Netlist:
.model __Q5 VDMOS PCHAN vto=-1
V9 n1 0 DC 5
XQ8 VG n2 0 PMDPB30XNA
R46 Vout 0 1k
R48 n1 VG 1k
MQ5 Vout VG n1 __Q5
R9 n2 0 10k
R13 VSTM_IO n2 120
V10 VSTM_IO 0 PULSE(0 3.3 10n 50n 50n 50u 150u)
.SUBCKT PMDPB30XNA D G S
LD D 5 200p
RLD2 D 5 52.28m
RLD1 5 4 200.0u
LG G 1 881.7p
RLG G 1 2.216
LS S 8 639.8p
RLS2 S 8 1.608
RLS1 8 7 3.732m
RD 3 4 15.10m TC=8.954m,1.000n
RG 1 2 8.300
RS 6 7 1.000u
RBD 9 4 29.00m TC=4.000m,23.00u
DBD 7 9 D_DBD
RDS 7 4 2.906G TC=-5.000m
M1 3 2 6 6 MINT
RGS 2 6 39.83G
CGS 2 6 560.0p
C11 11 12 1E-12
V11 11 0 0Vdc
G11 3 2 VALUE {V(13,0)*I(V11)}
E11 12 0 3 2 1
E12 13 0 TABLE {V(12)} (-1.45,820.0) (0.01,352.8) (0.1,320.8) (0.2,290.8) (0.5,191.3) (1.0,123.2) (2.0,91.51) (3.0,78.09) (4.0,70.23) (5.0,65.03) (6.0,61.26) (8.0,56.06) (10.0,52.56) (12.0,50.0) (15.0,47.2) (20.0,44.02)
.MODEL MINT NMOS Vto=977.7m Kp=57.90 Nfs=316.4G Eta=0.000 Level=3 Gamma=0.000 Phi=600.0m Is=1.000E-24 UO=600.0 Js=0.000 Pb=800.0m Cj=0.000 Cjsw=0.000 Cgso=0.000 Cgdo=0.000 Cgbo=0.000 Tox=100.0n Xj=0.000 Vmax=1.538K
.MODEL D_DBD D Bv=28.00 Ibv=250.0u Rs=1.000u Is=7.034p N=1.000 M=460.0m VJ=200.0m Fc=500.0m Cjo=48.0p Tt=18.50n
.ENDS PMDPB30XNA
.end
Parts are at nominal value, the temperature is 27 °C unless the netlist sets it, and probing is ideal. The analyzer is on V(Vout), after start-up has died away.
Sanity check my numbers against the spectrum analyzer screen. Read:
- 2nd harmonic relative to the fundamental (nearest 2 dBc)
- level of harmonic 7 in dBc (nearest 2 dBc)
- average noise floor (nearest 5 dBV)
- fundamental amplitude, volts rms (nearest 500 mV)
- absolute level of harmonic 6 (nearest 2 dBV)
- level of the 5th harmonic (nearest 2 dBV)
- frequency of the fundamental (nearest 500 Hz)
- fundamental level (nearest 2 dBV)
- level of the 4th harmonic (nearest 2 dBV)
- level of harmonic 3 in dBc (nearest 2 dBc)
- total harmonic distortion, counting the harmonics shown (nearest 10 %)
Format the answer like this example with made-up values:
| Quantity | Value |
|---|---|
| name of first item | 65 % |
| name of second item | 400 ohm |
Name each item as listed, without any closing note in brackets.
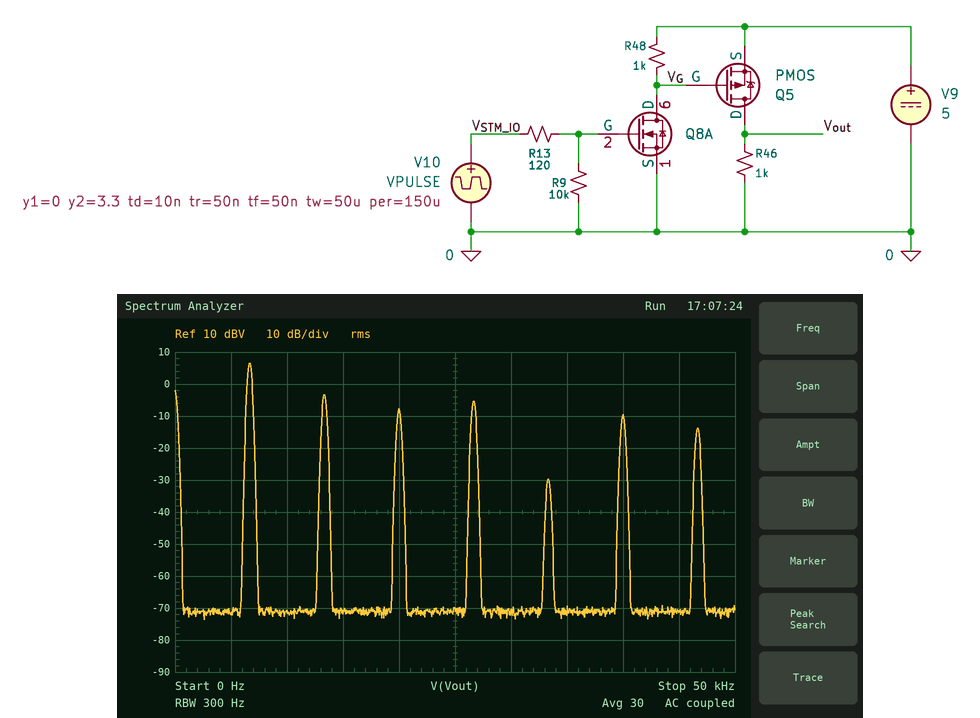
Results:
| Quantity | Value |
|---|---|
| 2nd harmonic relative to the fundamental | -10 dBc |
| level of harmonic 7 in dBc | -20 dBc |
| average noise floor | -70 dBV |
| fundamental amplitude, volts rms | 2.0 V |
| absolute level of harmonic 6 | -10 dBV |
| level of the 5th harmonic | -30 dBV |
| frequency of the fundamental | 6.5 kHz |
| fundamental level | 6 dBV |
| level of the 4th harmonic | -6 dBV |
| level of harmonic 3 in dBc | -14 dBc |
| total harmonic distortion, counting the harmonics shown | 50 % |
